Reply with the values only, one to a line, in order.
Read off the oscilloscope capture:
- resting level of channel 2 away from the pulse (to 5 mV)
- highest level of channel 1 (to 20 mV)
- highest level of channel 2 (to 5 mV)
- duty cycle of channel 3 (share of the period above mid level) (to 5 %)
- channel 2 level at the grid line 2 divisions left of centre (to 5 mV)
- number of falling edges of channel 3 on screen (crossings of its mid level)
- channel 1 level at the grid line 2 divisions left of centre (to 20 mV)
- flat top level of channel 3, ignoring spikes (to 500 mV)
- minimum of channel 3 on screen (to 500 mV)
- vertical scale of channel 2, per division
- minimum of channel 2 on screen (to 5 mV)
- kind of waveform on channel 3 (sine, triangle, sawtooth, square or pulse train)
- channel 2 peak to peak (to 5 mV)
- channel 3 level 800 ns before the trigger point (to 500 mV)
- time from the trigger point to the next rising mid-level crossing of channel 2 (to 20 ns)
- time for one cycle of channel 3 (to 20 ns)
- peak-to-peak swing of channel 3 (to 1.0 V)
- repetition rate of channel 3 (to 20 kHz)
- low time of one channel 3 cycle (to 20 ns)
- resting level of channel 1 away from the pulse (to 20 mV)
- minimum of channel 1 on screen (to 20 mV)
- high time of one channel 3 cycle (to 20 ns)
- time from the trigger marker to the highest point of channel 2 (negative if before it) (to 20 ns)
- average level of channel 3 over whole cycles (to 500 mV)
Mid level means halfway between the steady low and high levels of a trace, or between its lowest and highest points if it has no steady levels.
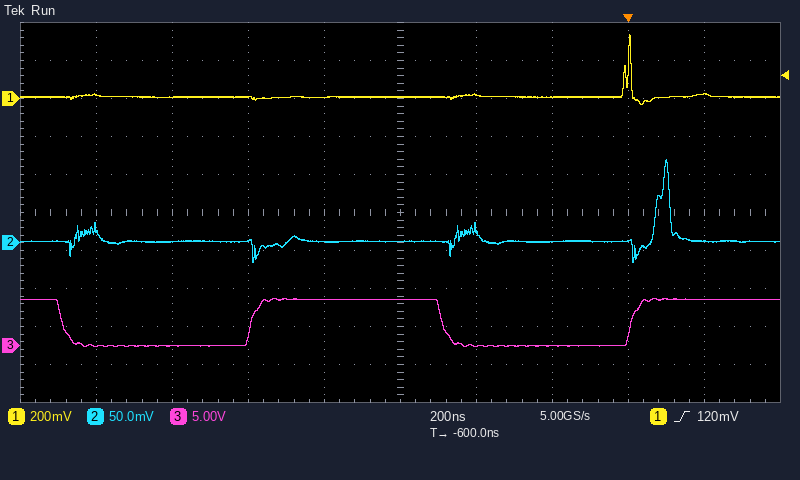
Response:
0 mV
340 mV
110 mV
50 %
0 mV
2
0 mV
6.0 V
0.0 V
50 mV
-25 mV
square
135 mV
6.0 V
80 ns
1.00 µs
6.0 V
1.00 MHz
500 ns
0 mV
-40 mV
500 ns
+100 ns
3.0 V
